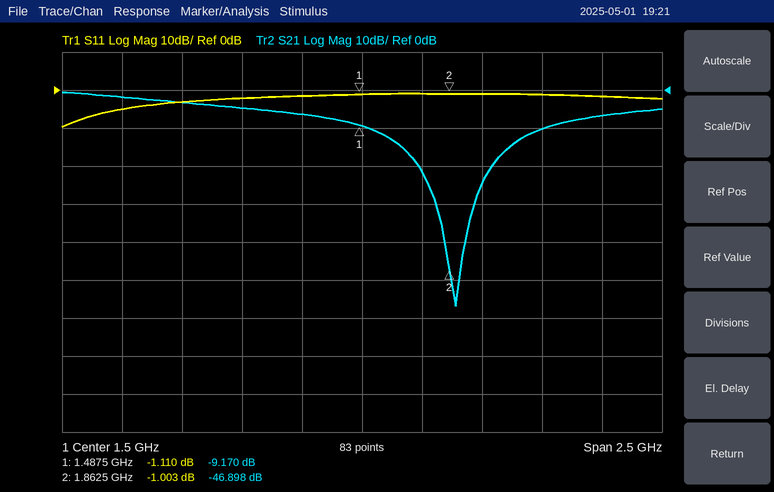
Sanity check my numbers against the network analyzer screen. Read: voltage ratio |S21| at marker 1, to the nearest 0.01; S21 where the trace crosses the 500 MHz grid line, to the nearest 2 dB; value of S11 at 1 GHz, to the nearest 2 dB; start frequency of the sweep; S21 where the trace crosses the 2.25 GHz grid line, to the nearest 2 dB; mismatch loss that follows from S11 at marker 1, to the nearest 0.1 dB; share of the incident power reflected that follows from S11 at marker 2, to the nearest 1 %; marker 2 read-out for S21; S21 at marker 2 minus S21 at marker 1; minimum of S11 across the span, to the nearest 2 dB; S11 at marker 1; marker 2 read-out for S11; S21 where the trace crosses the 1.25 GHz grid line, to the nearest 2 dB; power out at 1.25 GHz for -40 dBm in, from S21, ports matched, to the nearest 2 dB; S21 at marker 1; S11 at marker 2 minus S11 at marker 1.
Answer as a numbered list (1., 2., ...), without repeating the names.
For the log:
1. 0.35
2. -2 dB
3. -2 dB
4. 250 MHz
5. -10 dB
6. 6.5 dB
7. 79 %
8. -46.898 dB
9. -37.728 dB
10. -10 dB
11. -1.110 dB
12. -1.003 dB
13. -6 dB
14. -46 dBm
15. -9.170 dB
16. 0.107 dB
